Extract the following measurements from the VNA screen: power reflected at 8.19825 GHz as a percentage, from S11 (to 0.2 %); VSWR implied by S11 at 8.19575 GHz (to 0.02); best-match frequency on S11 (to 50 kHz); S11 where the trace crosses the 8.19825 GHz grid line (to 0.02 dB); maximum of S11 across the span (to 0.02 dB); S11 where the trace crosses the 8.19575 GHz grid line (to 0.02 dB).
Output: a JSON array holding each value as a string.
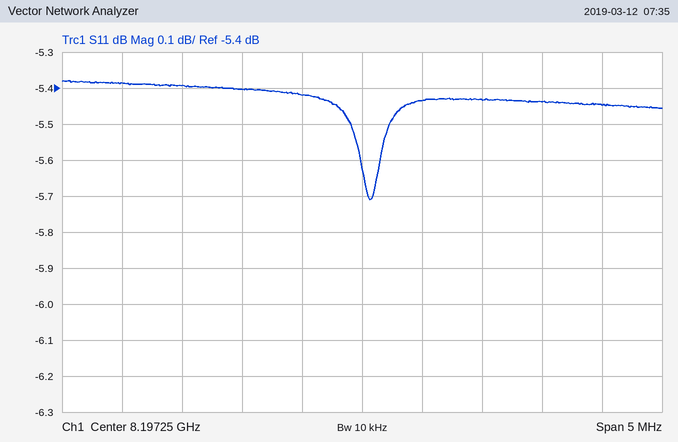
["28.6 %", "3.32", "8.19730 GHz", "-5.44 dB", "-5.38 dB", "-5.40 dB"]
